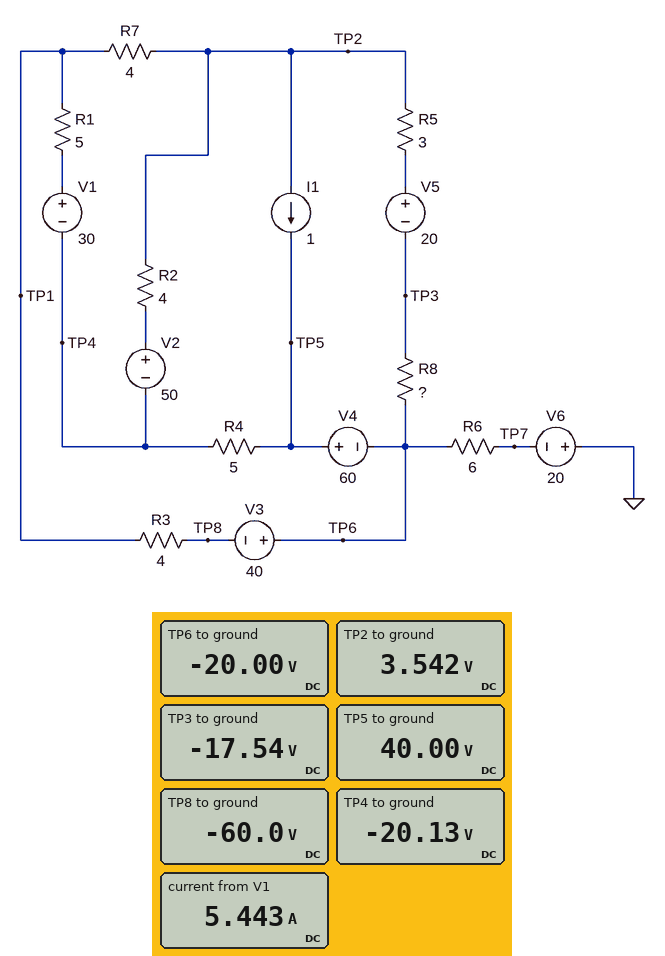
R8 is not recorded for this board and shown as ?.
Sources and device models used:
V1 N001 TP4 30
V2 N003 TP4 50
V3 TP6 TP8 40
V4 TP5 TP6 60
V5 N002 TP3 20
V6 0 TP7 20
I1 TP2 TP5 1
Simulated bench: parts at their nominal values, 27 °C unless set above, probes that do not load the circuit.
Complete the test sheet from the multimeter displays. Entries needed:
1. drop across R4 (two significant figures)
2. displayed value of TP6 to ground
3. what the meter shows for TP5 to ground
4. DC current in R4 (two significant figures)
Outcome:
60 V
-20.00 V
40.00 V
12 A
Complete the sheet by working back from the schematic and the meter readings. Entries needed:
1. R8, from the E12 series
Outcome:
6.8 Ω
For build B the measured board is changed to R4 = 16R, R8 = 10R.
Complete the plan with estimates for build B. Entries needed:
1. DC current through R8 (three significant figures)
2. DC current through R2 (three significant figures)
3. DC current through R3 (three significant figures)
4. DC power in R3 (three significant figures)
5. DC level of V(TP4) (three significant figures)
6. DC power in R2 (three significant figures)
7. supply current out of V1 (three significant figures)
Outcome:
1.42 A
3.66 A
6.29 A
158 W
-53.8 V
53.7 W
2.20 A
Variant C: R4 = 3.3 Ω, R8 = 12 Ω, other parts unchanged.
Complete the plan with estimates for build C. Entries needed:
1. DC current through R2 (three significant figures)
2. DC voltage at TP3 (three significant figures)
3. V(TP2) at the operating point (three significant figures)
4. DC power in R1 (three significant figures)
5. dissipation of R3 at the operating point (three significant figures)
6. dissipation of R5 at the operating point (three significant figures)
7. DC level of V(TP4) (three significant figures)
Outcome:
7.59 A
-9.90 V
12.6 V
222 W
616 W
2.12 W
-7.03 V
